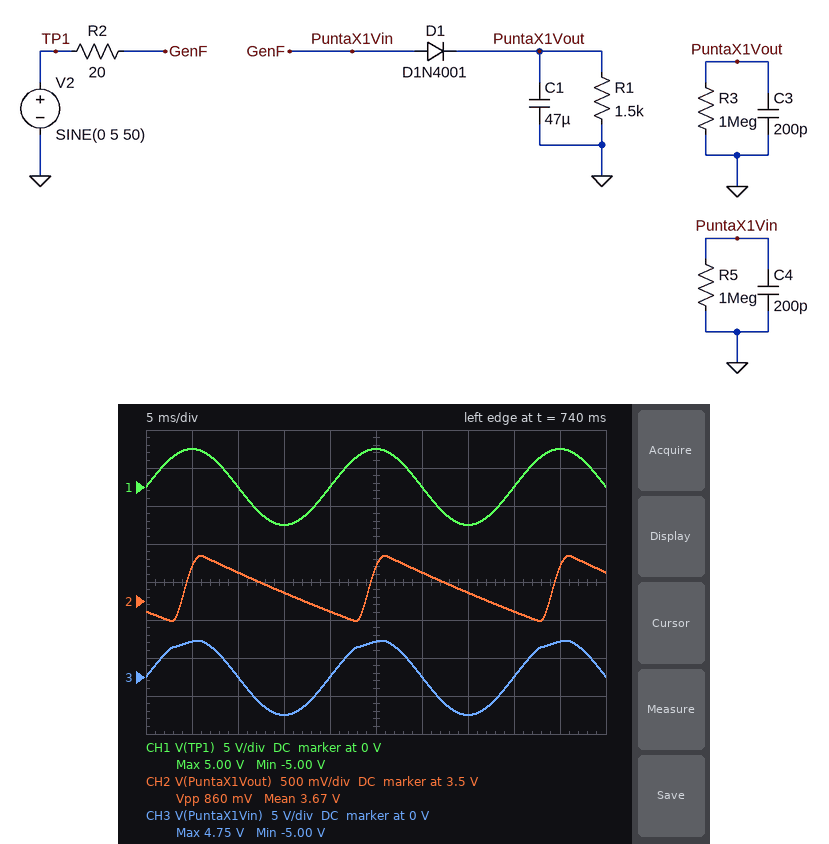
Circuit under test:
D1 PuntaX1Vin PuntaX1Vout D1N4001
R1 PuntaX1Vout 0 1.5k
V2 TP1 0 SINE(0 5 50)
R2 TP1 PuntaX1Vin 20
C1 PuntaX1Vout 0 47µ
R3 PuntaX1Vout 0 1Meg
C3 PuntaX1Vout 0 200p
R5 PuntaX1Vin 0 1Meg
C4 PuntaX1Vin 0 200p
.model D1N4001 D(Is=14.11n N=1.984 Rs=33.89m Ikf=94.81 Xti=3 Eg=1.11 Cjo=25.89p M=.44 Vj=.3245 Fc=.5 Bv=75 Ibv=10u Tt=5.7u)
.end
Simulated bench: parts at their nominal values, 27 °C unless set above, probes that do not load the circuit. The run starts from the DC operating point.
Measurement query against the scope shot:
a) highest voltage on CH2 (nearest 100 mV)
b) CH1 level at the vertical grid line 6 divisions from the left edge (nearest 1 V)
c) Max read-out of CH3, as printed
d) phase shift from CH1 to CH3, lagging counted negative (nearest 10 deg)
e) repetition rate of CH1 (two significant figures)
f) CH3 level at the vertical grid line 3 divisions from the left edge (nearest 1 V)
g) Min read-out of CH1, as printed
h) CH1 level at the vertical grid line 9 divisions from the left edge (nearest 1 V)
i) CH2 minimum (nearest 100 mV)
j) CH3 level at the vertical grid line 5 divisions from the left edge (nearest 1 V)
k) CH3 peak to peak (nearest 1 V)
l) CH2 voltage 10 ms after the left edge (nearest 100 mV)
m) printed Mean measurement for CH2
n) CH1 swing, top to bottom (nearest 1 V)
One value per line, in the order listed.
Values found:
4.1 V
0 V
4.75 V
0 deg
50 Hz
-5 V
-5.00 V
5 V
3.2 V
5 V
10 V
3.9 V
3.67 V
10 V
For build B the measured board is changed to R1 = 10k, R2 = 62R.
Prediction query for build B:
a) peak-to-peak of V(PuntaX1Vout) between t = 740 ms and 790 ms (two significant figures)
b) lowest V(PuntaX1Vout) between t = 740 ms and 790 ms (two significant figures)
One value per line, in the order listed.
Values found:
150 mV
4.0 V
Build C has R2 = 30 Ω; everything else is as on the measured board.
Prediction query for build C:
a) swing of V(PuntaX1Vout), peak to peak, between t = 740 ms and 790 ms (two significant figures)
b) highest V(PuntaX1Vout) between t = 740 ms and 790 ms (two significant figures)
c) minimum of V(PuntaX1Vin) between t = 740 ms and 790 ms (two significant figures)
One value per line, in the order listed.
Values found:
820 mV
4.0 V
-5.0 V
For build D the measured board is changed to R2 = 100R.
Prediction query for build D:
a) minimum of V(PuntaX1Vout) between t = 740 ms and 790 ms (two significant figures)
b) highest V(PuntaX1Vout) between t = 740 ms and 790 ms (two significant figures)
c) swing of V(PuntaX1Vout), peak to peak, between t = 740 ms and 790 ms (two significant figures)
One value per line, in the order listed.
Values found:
2.7 V
3.3 V
650 mV
